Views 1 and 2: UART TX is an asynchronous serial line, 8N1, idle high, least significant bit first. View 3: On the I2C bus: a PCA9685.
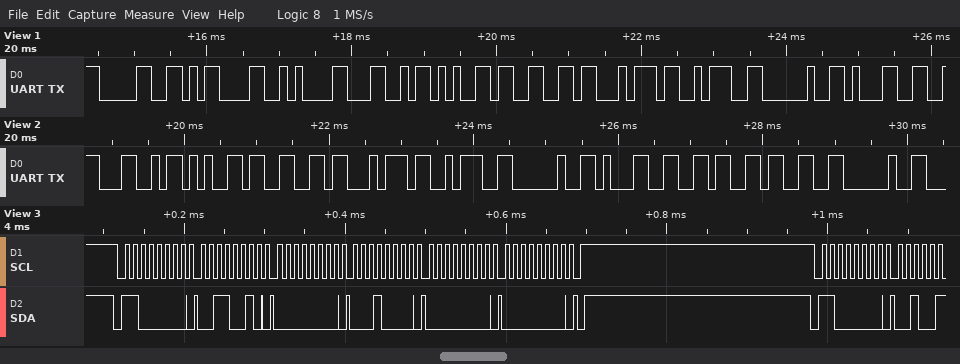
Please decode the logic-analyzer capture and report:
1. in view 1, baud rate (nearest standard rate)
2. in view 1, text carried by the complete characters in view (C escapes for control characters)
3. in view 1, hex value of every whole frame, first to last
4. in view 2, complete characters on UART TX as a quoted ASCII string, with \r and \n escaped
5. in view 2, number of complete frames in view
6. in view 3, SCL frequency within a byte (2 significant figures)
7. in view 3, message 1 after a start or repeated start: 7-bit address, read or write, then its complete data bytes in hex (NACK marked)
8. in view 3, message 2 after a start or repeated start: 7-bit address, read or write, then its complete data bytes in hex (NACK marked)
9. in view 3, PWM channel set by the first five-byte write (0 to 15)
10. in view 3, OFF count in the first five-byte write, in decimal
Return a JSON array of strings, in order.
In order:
["9600 baud", "\"0\\r\\nLeft: 1\"", "0x30 0x0D 0x0A 0x4C 0x65 0x66 0x74 0x3A 0x20 0x31", "\"Left: 163 \"", "10", "100 kHz", "0x60 write: 32 00 10 00 00", "0x60 write", "11", "0"]
